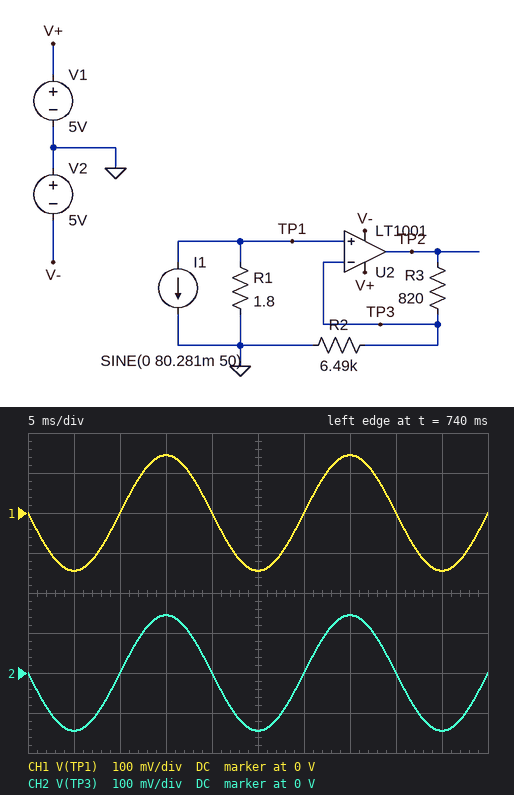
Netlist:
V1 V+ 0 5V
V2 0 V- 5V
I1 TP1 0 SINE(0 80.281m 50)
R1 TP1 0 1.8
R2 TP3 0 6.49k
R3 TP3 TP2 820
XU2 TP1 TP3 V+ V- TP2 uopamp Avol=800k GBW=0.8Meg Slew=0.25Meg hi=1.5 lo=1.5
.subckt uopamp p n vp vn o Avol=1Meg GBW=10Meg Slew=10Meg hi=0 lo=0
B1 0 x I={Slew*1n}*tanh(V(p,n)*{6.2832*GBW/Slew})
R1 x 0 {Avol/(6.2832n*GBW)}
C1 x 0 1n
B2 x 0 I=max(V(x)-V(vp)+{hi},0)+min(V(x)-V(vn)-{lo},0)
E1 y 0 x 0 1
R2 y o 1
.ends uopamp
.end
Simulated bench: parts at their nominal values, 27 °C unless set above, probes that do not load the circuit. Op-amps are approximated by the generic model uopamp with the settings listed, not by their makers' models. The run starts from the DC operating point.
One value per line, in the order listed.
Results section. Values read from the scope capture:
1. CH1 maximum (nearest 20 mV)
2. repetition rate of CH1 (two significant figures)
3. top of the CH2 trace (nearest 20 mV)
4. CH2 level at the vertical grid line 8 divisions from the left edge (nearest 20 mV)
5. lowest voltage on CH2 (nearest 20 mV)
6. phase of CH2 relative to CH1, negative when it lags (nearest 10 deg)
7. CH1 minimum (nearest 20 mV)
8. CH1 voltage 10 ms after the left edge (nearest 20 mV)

140 mV
50 Hz
140 mV
0 V
-140 mV
0 deg
-140 mV
0 V
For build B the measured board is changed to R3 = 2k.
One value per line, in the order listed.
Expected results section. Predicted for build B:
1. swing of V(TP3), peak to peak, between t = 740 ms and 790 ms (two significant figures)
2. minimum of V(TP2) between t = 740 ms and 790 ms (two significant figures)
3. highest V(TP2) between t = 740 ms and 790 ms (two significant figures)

290 mV
-190 mV
190 mV
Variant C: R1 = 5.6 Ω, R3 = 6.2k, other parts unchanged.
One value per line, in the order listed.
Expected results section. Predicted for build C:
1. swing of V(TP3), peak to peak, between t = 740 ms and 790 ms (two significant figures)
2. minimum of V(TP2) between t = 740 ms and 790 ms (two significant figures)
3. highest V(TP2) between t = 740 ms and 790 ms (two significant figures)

900 mV
-880 mV
880 mV
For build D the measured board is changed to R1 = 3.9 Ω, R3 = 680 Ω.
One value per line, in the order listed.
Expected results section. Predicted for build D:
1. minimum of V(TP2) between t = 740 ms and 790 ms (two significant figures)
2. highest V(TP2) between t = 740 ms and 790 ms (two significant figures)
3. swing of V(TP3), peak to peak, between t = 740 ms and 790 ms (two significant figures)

-350 mV
350 mV
630 mV
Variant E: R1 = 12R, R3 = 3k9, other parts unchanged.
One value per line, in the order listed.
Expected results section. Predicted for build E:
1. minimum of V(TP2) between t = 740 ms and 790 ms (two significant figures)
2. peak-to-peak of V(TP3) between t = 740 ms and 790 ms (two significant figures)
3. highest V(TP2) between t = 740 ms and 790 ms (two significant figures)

-1.5 V
1.9 V
1.5 V
